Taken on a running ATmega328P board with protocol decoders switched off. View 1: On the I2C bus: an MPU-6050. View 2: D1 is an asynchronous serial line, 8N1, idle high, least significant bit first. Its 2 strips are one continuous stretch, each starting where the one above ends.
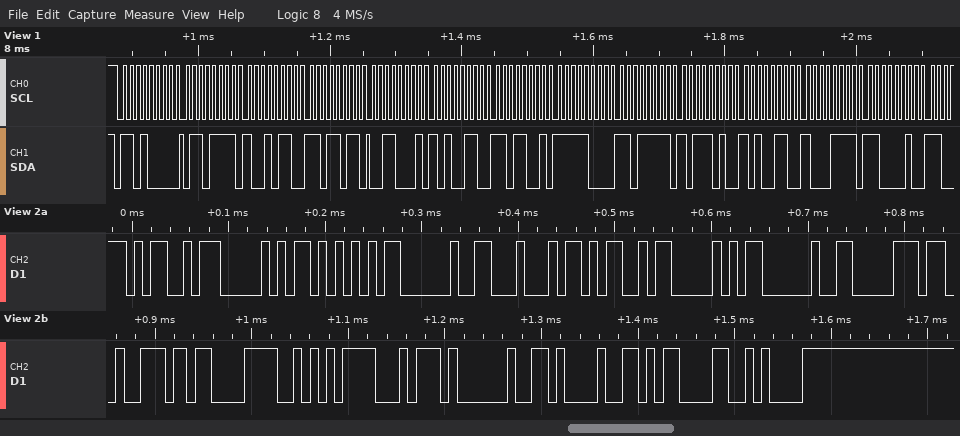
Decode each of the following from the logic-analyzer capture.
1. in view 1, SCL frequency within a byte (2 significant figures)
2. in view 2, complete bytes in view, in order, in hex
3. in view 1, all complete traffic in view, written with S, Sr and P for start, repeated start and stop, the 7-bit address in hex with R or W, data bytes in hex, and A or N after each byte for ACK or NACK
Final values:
100 kHz
4D 50 55 20 44 4D 50 20 70 72 C3 AA 74 20 21 0D 0A
S 68W A 6F A 96 A DB A 31 A A6 A D9 A F8 A DF A BA A A6 A 8F A C2 A
